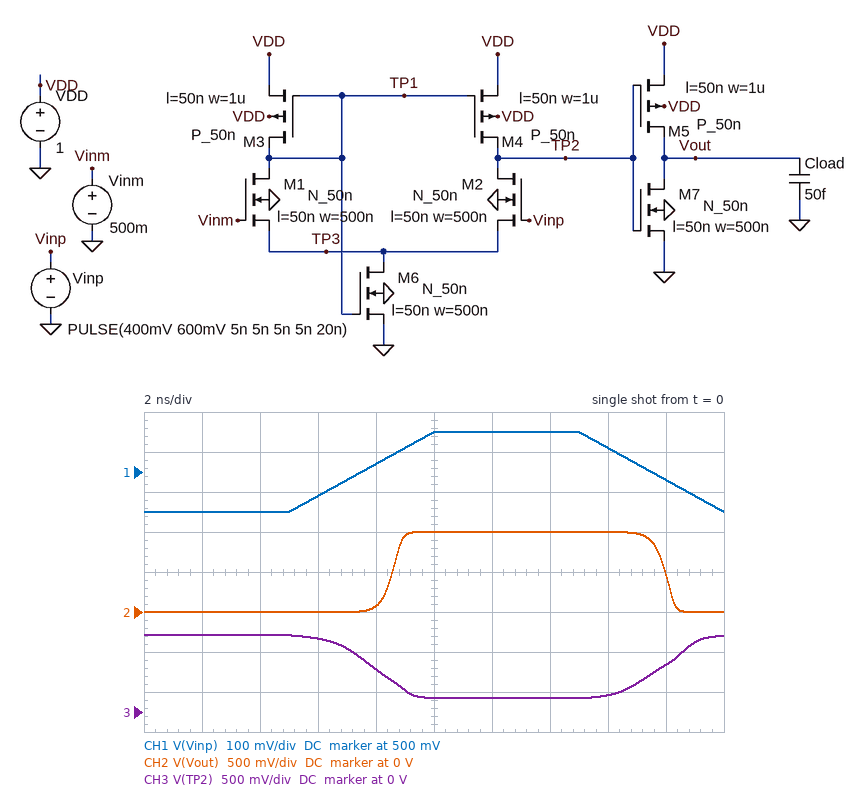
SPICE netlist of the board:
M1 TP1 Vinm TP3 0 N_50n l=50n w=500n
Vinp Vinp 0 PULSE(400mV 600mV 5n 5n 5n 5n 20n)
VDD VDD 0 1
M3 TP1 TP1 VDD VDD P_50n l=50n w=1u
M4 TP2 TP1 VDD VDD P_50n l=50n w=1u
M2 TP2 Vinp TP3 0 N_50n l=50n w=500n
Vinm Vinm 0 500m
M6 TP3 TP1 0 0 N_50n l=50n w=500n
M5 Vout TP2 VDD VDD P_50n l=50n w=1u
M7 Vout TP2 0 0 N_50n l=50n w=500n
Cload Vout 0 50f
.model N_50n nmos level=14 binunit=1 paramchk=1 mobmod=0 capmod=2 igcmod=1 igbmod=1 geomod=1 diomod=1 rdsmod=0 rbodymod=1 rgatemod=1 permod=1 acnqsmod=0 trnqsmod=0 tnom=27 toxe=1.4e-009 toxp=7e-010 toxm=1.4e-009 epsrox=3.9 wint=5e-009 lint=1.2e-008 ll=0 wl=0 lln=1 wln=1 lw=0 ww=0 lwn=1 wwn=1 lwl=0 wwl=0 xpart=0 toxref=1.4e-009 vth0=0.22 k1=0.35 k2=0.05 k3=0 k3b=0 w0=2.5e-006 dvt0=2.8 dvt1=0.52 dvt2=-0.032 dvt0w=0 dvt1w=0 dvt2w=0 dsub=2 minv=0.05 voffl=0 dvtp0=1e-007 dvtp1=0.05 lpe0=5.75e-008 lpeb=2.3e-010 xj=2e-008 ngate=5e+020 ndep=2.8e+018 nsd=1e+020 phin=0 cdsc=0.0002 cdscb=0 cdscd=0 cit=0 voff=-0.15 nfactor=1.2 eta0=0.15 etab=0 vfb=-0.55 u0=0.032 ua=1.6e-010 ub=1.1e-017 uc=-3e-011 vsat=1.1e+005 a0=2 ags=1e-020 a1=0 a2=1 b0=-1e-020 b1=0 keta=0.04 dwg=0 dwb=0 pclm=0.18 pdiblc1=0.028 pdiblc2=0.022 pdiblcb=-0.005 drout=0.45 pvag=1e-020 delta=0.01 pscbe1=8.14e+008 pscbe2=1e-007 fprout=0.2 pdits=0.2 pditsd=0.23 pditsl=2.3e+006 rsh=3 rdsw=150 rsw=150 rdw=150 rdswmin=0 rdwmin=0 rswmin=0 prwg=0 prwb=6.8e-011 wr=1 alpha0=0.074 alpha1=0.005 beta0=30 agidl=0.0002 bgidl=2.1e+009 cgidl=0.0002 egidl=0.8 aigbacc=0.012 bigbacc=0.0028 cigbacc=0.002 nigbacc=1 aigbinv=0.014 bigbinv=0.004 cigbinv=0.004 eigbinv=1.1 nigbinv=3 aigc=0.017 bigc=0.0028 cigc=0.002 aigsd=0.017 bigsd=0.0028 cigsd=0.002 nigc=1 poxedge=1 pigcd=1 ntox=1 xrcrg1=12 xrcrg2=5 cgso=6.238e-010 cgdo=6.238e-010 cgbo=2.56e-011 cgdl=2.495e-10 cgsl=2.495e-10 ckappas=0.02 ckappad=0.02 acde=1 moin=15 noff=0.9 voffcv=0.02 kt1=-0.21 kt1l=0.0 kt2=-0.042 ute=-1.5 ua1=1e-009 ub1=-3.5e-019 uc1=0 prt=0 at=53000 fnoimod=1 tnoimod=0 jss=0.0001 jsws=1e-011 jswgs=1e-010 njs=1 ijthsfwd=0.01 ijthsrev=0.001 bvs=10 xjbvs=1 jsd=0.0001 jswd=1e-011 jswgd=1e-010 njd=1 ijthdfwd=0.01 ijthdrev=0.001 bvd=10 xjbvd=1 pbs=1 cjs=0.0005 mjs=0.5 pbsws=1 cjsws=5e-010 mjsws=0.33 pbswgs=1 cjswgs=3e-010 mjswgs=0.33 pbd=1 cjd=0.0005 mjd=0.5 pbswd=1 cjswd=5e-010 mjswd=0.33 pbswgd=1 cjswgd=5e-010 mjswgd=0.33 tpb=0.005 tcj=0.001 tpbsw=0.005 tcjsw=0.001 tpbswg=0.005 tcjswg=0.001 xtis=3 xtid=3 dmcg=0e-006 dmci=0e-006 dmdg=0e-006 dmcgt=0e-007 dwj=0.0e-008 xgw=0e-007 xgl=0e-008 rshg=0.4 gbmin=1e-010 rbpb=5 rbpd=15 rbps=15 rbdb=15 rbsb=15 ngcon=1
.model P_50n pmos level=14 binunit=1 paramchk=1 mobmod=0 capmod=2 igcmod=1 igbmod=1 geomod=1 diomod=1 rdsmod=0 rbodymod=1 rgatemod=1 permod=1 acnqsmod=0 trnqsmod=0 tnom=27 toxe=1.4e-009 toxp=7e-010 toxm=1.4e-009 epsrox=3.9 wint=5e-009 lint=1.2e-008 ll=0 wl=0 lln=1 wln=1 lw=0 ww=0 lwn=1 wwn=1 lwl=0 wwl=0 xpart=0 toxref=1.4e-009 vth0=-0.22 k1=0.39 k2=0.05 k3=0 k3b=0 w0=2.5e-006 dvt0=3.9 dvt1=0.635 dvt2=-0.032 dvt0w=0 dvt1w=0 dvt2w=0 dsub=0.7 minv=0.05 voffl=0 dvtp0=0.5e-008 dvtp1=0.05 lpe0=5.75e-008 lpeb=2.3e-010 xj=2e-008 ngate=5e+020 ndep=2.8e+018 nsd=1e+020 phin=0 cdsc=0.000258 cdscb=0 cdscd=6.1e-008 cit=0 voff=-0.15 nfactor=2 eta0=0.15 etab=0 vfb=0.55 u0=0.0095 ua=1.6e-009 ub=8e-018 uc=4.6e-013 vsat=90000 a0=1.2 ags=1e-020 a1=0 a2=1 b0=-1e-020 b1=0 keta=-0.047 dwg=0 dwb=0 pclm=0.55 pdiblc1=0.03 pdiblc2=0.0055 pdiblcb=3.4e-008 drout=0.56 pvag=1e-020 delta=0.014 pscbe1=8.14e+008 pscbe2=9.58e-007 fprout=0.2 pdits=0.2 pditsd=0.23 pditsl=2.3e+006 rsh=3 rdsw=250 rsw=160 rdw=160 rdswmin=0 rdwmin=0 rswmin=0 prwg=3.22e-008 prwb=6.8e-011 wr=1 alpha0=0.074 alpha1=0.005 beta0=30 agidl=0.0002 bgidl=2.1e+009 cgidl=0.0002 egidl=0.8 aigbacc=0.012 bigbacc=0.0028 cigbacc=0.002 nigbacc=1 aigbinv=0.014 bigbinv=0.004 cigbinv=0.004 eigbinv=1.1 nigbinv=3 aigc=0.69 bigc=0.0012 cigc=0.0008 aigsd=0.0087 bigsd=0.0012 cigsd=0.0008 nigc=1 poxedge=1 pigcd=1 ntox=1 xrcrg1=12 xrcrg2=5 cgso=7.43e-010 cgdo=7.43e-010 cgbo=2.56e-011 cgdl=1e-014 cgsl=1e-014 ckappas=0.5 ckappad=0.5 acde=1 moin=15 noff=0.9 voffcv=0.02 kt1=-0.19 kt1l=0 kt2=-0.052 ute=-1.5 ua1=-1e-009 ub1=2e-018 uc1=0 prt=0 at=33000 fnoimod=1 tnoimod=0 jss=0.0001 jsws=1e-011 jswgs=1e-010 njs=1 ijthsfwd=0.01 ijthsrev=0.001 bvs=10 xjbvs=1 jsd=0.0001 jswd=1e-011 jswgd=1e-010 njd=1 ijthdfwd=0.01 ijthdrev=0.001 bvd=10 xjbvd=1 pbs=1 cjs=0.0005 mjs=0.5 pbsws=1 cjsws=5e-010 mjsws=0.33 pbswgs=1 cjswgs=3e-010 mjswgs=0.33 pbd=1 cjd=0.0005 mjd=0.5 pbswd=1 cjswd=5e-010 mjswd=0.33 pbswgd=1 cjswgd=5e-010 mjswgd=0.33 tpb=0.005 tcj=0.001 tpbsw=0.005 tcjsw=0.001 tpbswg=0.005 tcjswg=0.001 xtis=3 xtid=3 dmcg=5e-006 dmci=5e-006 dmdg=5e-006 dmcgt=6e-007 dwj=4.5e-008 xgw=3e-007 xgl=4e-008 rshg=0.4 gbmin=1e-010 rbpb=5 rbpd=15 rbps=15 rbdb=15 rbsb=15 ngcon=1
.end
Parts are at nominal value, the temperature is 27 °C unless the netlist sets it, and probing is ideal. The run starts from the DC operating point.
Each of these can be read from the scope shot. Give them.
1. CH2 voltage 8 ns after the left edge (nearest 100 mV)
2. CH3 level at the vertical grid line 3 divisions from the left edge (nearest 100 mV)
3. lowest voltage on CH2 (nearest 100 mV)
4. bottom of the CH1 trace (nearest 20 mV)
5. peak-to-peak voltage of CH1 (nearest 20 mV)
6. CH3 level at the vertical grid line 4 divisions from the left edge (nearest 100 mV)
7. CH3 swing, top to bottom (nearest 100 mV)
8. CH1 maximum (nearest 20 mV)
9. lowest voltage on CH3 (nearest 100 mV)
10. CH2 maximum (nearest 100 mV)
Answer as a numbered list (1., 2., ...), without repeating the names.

1. 100 mV
2. 900 mV
3. 0 V
4. 400 mV
5. 200 mV
6. 500 mV
7. 800 mV
8. 600 mV
9. 200 mV
10. 1.0 V
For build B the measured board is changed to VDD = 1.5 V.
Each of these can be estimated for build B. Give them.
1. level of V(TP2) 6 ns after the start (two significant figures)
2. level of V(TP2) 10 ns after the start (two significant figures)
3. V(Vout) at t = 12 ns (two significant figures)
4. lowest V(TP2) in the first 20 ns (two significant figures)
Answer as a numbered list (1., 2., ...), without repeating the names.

1. 1.4 V
2. 390 mV
3. 1.5 V
4. 350 mV
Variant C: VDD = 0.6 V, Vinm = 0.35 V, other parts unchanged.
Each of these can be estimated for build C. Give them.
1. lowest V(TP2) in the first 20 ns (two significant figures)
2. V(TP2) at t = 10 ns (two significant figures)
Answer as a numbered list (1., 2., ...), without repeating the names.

1. 82 mV
2. 83 mV
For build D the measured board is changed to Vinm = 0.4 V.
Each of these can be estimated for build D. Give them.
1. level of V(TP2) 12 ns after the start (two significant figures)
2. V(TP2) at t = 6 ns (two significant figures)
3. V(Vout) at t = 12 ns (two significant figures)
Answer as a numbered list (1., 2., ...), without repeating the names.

1. 79 mV
2. 450 mV
3. 1.0 V
